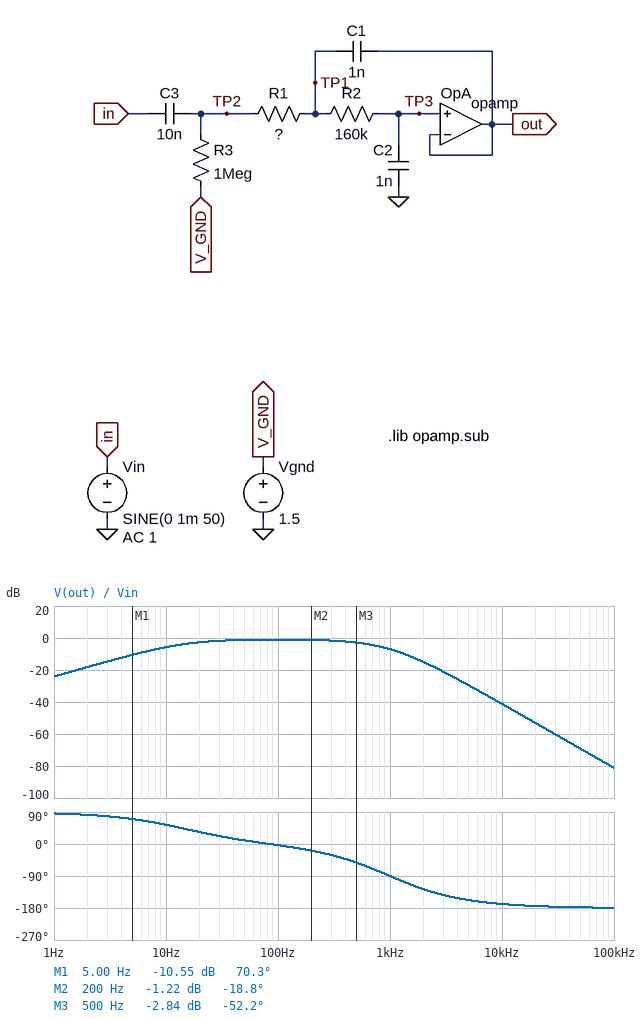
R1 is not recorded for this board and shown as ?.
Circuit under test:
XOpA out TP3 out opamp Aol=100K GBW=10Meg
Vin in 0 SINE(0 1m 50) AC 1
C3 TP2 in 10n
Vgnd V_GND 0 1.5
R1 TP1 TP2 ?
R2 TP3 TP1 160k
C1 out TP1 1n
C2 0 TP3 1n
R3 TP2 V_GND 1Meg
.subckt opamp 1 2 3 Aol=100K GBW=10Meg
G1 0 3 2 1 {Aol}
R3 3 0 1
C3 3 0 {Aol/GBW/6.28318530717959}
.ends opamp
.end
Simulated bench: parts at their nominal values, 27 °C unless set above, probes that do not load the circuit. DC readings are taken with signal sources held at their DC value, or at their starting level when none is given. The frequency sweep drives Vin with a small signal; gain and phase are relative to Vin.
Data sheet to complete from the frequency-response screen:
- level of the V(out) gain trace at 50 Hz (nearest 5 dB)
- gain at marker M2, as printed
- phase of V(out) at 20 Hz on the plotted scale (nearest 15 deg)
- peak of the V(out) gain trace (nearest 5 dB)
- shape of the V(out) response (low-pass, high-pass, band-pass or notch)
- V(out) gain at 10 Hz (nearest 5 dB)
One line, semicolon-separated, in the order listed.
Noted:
0 dB; -1.22 dB; 30 deg; 0 dB; band-pass; -5 dB
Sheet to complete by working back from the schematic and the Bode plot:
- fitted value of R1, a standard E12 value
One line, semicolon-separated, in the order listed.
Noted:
180 kΩ
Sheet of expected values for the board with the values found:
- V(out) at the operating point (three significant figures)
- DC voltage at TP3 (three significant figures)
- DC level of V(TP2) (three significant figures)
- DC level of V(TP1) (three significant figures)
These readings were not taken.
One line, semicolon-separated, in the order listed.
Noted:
1.50 V; 1.50 V; 1.50 V; 1.50 V
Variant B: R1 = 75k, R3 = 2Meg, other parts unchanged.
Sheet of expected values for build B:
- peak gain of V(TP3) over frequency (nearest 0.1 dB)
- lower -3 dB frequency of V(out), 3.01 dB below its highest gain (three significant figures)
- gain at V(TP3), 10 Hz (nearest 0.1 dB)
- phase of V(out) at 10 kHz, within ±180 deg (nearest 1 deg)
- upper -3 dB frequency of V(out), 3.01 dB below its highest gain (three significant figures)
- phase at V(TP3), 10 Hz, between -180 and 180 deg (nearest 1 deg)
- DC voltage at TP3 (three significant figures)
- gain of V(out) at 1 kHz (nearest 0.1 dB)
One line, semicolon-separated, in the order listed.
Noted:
-0.9 dB; 7.12 Hz; -2.7 dB; -161 deg; 878 Hz; 35 deg; 1.50 V; -4.6 dB
